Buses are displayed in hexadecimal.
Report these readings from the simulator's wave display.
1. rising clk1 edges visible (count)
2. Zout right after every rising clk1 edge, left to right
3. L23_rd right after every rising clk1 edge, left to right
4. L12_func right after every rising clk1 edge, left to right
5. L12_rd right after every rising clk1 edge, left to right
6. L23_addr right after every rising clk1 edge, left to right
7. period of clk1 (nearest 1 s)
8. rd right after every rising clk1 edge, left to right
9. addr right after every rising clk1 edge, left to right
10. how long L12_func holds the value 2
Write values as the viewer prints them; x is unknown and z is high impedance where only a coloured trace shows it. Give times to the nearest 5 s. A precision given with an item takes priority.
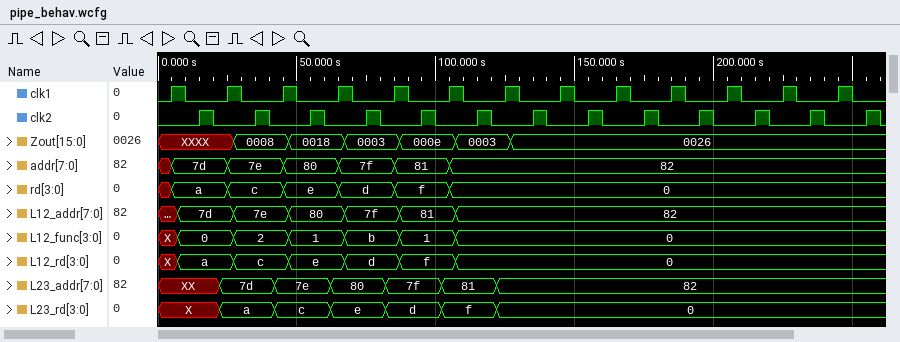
13
XXXX, XXXX, 0008, 0018, 0003, 000e, 0003, 0026, 0026, 0026, 0026, 0026, 0026
X, a, c, e, d, f, 0, 0, 0, 0, 0, 0, 0
X, 0, 2, 1, b, 1, 0, 0, 0, 0, 0, 0, 0
X, a, c, e, d, f, 0, 0, 0, 0, 0, 0, 0
XX, 7d, 7e, 80, 7f, 81, 82, 82, 82, 82, 82, 82, 82
20 s
a, c, e, d, f, 0, 0, 0, 0, 0, 0, 0, 0
7d, 7e, 80, 7f, 81, 82, 82, 82, 82, 82, 82, 82, 82
20 s
